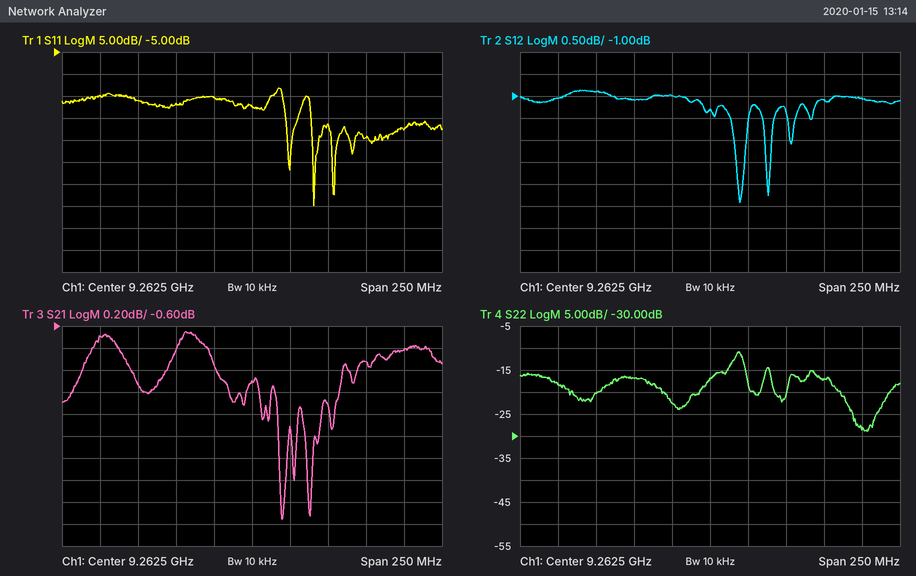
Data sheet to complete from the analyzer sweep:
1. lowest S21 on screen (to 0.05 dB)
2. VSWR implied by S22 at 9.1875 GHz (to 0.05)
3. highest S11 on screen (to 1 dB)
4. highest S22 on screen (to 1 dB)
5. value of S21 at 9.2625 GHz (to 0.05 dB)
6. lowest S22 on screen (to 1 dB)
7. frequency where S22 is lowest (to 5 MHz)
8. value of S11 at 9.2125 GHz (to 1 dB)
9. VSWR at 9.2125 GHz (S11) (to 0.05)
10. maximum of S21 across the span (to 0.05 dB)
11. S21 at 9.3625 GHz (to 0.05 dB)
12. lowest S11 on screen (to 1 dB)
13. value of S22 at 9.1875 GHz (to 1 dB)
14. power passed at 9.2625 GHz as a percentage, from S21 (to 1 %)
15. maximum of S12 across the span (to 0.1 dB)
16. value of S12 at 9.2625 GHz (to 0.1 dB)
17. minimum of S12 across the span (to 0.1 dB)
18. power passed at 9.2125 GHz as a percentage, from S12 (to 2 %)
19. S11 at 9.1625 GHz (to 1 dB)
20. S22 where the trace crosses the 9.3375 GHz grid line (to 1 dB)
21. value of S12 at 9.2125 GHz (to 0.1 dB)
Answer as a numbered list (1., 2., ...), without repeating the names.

1. -2.35 dB
2. 1.20
3. -13 dB
4. -11 dB
5. -1.10 dB
6. -29 dB
7. 9.365 GHz
8. -17 dB
9. 1.35
10. -0.65 dB
11. -0.80 dB
12. -40 dB
13. -20 dB
14. 78 %
15. -0.9 dB
16. -1.3 dB
17. -3.4 dB
18. 78 %
19. -15 dB
20. -17 dB
21. -1.1 dB
